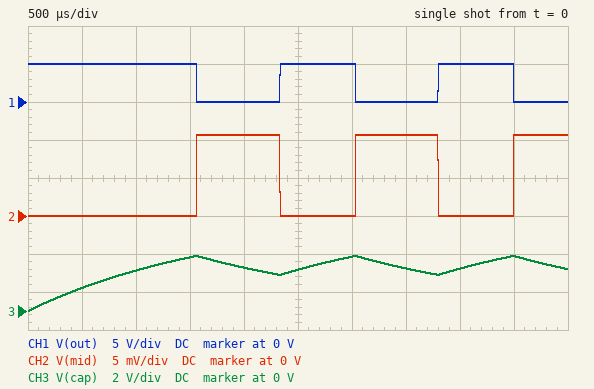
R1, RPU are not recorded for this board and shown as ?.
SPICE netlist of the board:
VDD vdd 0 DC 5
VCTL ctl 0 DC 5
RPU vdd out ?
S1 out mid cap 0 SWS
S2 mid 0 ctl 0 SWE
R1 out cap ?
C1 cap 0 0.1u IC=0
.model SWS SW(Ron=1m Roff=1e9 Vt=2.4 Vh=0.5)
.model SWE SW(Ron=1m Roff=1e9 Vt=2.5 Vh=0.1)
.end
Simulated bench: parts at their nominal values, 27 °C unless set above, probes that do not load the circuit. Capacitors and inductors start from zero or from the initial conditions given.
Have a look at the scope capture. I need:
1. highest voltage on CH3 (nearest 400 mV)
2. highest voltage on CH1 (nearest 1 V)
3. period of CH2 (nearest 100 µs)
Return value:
2.8 V
5 V
1.5 ms
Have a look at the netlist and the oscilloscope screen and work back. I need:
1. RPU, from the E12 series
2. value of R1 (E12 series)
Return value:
0.47 Ω
18 kΩ
